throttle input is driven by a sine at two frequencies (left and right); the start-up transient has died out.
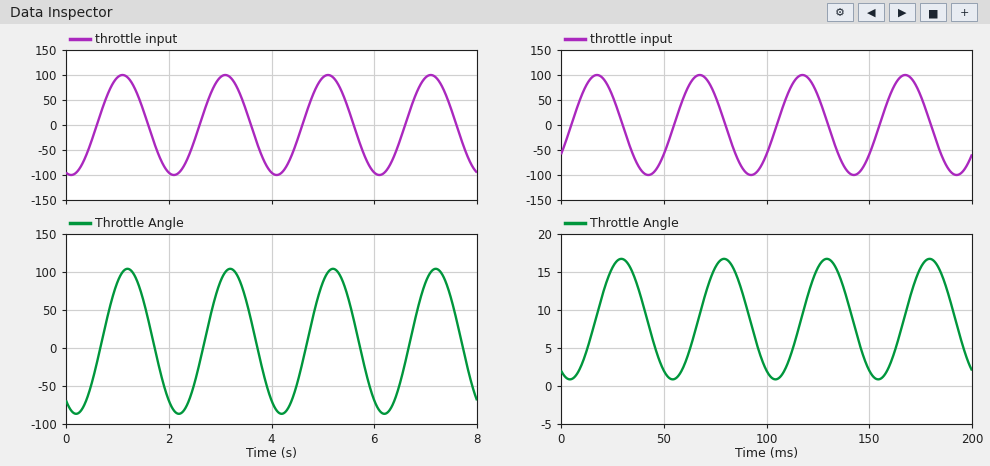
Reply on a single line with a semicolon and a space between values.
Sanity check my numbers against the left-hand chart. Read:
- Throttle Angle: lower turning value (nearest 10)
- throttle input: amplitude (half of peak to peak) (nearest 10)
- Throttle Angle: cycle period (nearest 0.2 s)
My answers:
-90; 100; 2.0 s
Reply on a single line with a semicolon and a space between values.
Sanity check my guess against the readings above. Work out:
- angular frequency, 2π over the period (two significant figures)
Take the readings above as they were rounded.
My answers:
3.1 rad/s
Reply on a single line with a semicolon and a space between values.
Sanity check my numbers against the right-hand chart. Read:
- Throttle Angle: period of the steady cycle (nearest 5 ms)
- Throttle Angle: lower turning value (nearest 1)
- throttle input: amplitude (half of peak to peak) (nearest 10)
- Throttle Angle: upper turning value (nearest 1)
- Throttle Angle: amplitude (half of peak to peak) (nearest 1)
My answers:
50 ms; 1; 100; 17; 8
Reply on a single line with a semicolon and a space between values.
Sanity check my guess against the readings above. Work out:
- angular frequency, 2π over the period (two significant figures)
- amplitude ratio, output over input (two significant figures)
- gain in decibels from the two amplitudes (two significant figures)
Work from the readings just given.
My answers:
0.13 rad/ms; 0.080; -22 dB
